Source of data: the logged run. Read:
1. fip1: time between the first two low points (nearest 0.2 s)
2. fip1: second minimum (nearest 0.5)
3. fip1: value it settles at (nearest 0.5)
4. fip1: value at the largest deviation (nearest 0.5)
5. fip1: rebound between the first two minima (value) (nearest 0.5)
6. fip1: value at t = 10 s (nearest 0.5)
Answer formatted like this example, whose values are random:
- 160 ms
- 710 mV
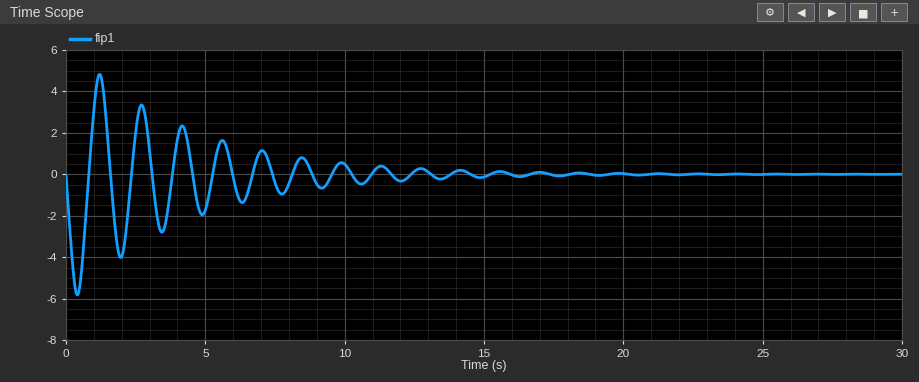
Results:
- 1.6 s
- -4.0
- 0.0
- -6.0
- 5.0
- 0.5
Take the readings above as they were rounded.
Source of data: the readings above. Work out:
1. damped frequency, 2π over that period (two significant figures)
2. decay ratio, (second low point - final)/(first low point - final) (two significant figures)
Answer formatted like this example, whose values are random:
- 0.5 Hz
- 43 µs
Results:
- 3.9 rad/s
- 0.67
